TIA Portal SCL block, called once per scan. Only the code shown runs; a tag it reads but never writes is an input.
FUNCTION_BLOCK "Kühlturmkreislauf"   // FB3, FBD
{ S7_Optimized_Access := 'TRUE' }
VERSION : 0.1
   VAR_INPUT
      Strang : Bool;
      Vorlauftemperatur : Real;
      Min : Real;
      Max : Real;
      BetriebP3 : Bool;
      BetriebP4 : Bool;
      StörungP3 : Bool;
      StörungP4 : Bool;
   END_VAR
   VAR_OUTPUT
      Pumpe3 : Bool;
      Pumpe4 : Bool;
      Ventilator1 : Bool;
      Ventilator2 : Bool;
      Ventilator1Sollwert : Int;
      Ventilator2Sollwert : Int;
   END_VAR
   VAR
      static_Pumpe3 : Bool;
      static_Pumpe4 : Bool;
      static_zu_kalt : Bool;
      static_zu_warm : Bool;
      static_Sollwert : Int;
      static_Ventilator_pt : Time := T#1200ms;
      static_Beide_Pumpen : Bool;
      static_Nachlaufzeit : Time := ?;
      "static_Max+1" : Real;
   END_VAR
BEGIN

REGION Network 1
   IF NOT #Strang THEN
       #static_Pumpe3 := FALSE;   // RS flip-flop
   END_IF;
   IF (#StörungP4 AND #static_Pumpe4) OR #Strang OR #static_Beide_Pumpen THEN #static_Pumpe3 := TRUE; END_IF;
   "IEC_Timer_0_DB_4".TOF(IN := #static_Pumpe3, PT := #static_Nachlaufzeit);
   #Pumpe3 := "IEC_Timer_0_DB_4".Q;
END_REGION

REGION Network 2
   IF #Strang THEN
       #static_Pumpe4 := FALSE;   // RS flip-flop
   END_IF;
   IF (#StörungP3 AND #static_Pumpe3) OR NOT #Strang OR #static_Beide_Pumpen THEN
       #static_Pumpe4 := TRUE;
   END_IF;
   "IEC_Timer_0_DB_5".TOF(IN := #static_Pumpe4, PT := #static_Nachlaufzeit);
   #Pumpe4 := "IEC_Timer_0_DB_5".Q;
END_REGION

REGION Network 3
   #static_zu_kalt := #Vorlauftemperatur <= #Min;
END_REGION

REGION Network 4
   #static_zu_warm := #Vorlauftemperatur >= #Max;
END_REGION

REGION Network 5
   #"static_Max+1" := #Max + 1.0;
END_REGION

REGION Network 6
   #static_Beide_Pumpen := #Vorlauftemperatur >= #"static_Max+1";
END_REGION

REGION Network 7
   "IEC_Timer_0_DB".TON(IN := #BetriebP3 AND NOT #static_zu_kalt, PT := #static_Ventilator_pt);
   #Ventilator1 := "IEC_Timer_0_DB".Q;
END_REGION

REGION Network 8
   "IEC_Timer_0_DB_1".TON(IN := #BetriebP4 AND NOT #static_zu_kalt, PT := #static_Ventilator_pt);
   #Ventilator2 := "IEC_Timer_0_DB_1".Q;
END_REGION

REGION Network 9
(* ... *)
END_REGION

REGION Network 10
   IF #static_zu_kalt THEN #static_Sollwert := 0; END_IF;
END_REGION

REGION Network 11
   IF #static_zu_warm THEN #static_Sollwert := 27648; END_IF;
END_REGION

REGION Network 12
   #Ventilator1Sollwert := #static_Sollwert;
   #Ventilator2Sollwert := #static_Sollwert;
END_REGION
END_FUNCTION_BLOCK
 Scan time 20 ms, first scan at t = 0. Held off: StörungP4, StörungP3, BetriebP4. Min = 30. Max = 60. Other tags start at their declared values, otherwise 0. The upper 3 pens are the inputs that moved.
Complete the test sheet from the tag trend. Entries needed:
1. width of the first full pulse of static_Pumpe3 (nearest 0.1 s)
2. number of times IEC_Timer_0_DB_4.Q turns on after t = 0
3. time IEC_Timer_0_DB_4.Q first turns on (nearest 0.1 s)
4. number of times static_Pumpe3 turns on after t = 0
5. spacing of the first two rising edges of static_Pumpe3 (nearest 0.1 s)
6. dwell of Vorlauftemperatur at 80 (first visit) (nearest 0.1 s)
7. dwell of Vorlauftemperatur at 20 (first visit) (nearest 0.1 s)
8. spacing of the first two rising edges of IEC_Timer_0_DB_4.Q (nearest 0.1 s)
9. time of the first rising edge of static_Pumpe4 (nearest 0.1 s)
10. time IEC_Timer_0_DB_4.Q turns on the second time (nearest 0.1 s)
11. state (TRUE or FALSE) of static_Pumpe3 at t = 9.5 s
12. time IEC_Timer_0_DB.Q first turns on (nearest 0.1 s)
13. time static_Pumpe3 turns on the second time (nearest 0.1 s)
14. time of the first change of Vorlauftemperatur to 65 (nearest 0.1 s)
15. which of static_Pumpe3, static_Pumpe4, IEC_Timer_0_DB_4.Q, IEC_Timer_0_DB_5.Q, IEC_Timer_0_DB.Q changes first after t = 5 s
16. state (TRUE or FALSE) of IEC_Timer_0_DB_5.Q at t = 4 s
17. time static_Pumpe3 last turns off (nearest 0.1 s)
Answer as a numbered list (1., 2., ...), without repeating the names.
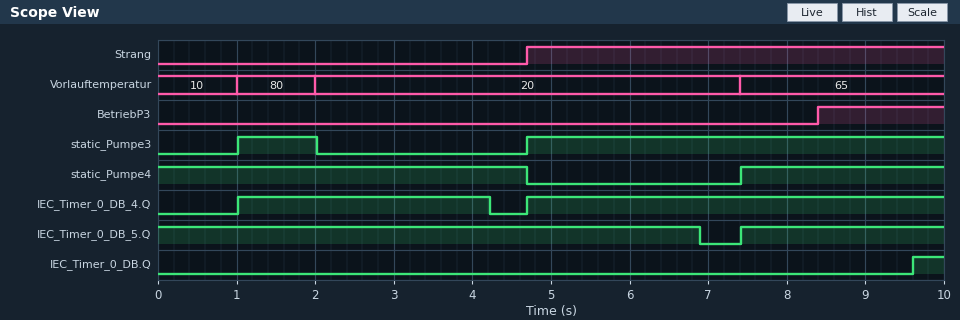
1. 1.0 s
2. 2
3. 1.0 s
4. 2
5. 3.7 s
6. 1.0 s
7. 5.4 s
8. 3.7 s
9. 7.4 s
10. 4.7 s
11. TRUE
12. 9.6 s
13. 4.7 s
14. 7.4 s
15. IEC_Timer_0_DB_5.Q
16. TRUE
17. 2.0 s
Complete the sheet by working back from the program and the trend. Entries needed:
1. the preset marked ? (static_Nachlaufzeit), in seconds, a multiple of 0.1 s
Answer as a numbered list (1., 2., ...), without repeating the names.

1. 2.2 s
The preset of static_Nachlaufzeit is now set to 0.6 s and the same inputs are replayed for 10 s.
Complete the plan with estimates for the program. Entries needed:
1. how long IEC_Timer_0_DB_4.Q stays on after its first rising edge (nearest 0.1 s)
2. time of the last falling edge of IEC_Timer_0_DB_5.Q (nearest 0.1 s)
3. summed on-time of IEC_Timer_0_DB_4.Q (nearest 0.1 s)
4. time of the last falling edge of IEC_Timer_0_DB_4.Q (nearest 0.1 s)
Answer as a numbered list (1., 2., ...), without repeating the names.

1. 1.6 s
2. 5.3 s
3. 6.9 s
4. 2.6 s
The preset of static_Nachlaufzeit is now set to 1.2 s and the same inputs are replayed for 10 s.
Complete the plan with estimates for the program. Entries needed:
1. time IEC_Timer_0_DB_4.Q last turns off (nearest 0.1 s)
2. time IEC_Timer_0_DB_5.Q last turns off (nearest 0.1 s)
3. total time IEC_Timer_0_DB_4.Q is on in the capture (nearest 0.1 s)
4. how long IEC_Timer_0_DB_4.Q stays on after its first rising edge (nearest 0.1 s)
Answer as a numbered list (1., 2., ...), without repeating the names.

1. 3.2 s
2. 5.9 s
3. 7.5 s
4. 2.2 s
